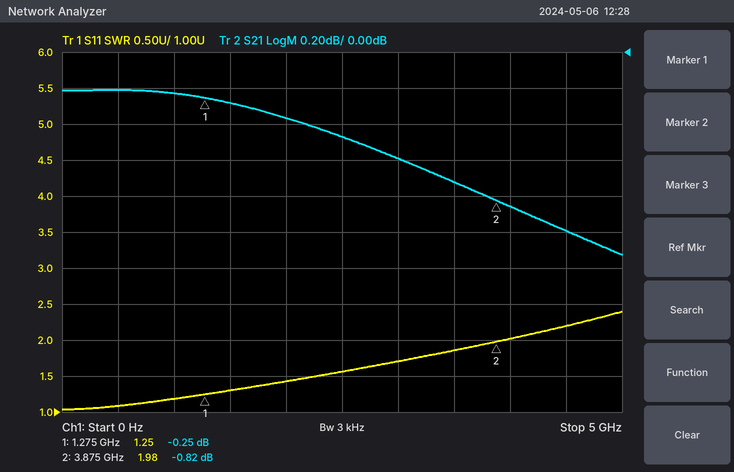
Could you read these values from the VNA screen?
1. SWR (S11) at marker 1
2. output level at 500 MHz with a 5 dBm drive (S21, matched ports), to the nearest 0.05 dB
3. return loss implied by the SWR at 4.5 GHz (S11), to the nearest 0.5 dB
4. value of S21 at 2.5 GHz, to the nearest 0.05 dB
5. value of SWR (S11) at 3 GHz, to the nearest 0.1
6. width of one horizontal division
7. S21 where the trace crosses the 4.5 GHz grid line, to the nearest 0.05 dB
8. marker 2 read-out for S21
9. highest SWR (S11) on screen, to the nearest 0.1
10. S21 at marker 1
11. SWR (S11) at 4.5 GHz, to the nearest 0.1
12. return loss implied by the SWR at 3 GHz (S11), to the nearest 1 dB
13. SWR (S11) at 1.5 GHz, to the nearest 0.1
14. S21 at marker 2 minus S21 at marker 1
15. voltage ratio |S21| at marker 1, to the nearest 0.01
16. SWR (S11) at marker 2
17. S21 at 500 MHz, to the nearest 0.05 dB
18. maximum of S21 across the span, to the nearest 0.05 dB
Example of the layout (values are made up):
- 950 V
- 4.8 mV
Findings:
- 1.25
- 4.80 dBm
- 8.5 dB
- -0.45 dB
- 1.7
- 500 MHz
- -1.00 dB
- -0.82 dB
- 2.4
- -0.25 dB
- 2.2
- 12 dB
- 1.3
- -0.57 dB
- 0.97
- 1.98
- -0.20 dB
- -0.20 dB
